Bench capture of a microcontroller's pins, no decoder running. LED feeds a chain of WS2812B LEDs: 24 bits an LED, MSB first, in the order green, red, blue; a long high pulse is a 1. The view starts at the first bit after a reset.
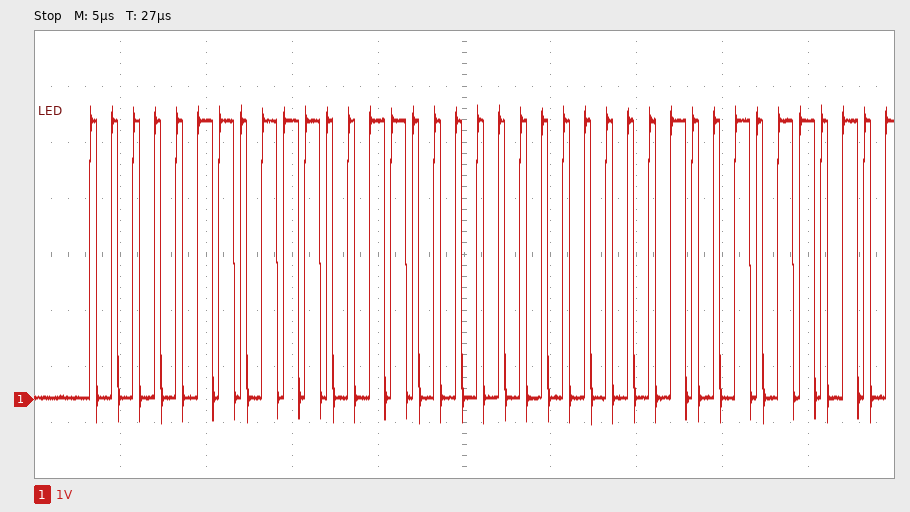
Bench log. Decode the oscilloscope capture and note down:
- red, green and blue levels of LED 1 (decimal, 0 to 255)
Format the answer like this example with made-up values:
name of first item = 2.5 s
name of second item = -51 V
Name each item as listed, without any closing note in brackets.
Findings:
red, green and blue levels of LED 1 = 230, 6, 0
